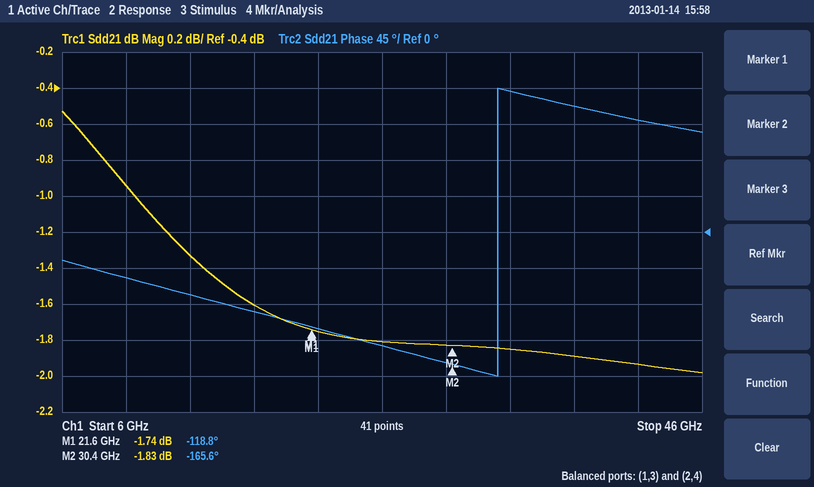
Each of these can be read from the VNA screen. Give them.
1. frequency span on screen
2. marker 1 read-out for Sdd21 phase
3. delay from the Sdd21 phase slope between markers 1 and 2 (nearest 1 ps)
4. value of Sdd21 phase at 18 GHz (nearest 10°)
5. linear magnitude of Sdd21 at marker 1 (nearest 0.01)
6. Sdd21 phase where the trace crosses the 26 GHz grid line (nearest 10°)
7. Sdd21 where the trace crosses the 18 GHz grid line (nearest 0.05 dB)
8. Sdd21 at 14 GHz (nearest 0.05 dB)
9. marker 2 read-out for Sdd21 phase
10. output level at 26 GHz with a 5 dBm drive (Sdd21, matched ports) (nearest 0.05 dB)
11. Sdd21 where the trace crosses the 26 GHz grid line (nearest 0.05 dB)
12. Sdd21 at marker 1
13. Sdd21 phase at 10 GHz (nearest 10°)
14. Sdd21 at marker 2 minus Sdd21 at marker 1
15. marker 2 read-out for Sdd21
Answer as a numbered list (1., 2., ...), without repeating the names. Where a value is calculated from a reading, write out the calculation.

1. 40 GHz
2. -118.8°
3. −(-165.6° − (-118.8°))/(360° × 8.8 GHz) ≈ 15 ps
4. -100°
5. 10^(-1.74/20) ≈ 0.82
6. -140°
7. -1.60 dB
8. -1.35 dB
9. -165.6°
10. 5 dBm + (-1.80 dB) = 3.20 dBm
11. -1.80 dB
12. -1.74 dB
13. -60°
14. -1.83 − (-1.74) = -0.09 dB
15. -1.83 dB
